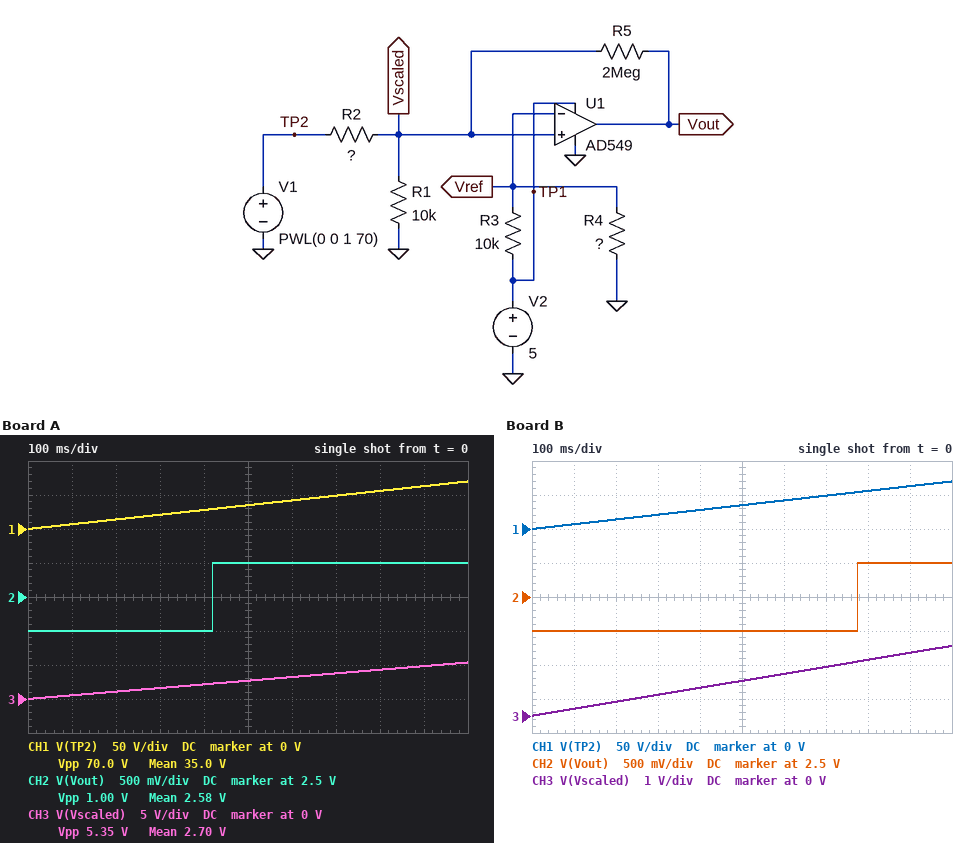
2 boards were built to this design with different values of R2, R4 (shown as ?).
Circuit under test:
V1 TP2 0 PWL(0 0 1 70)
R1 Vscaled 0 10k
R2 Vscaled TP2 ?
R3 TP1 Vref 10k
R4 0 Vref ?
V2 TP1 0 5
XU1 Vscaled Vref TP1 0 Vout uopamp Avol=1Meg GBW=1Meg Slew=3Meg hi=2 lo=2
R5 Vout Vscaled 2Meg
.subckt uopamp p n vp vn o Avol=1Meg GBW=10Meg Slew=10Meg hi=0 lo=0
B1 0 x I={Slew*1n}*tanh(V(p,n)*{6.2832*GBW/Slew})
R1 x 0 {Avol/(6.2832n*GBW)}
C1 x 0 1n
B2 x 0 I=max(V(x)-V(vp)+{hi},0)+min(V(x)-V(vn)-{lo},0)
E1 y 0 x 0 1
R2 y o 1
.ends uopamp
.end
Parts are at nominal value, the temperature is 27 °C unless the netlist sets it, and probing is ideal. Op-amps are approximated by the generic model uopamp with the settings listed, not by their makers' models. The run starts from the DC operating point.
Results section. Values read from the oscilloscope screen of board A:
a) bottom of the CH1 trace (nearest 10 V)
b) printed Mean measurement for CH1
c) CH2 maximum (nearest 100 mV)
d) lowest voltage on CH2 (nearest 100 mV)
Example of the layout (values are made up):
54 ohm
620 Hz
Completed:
0 V
35.0 V
3.0 V
2.0 V
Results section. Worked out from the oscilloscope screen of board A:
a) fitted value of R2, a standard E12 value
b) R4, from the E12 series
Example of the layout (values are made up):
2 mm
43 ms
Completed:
120 kΩ
8.2 kΩ
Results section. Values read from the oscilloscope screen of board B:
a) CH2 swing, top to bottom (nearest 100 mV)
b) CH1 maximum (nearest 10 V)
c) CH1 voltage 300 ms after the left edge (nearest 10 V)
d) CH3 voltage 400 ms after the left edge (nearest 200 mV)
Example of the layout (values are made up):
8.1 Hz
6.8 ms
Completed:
1.0 V
70 V
20 V
800 mV
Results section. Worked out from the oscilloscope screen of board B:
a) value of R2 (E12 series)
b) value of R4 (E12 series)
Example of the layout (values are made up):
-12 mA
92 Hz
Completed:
330 kΩ
4.7 kΩ
